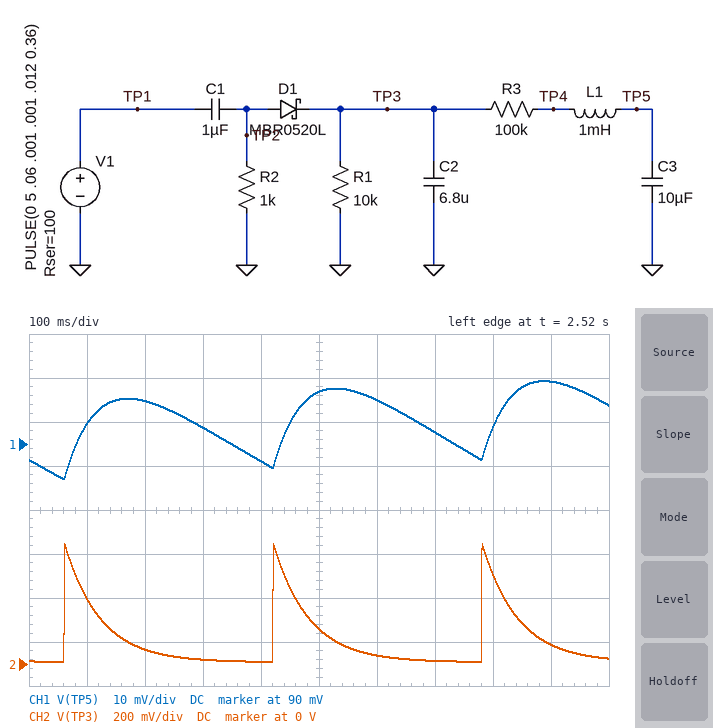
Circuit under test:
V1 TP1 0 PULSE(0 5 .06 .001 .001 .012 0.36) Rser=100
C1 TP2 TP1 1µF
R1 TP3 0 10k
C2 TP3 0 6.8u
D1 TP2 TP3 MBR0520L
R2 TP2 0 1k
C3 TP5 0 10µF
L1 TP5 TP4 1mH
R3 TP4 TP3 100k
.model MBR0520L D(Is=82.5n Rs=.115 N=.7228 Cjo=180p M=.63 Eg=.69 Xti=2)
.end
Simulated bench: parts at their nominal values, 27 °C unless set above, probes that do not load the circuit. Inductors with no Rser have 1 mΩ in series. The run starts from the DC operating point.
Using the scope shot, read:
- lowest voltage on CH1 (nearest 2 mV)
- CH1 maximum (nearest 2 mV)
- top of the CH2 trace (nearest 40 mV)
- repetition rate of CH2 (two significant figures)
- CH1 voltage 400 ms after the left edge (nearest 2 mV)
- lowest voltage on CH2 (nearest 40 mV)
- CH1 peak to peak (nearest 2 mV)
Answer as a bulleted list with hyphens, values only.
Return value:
- 82 mV
- 104 mV
- 560 mV
- 2.8 Hz
- 86 mV
- 0 V
- 22 mV
